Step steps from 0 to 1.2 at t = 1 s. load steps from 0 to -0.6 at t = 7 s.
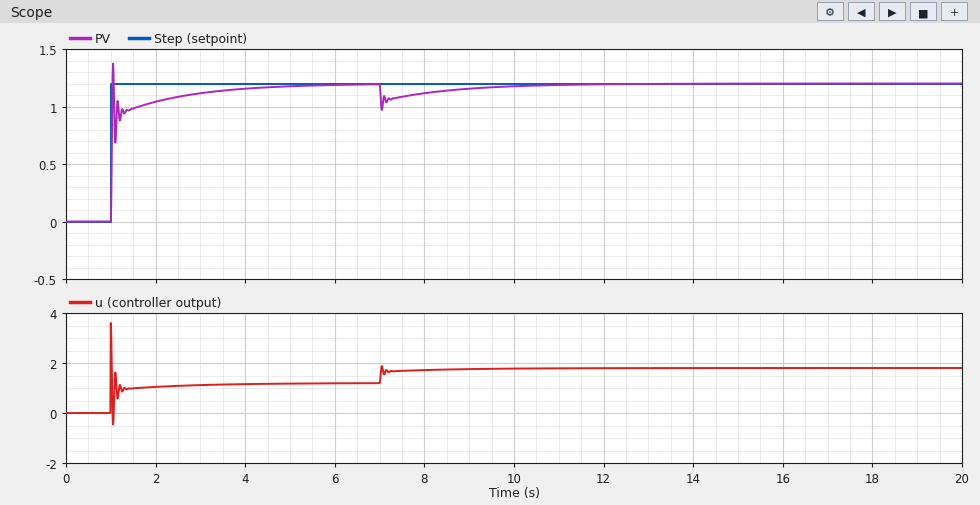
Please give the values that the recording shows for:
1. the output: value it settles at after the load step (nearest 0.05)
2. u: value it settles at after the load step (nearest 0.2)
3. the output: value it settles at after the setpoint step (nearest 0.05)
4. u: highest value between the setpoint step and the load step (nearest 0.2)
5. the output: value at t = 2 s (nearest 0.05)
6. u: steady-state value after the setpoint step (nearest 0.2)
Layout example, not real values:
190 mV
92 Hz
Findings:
1.20
1.8
1.20
3.6
1.05
1.2
